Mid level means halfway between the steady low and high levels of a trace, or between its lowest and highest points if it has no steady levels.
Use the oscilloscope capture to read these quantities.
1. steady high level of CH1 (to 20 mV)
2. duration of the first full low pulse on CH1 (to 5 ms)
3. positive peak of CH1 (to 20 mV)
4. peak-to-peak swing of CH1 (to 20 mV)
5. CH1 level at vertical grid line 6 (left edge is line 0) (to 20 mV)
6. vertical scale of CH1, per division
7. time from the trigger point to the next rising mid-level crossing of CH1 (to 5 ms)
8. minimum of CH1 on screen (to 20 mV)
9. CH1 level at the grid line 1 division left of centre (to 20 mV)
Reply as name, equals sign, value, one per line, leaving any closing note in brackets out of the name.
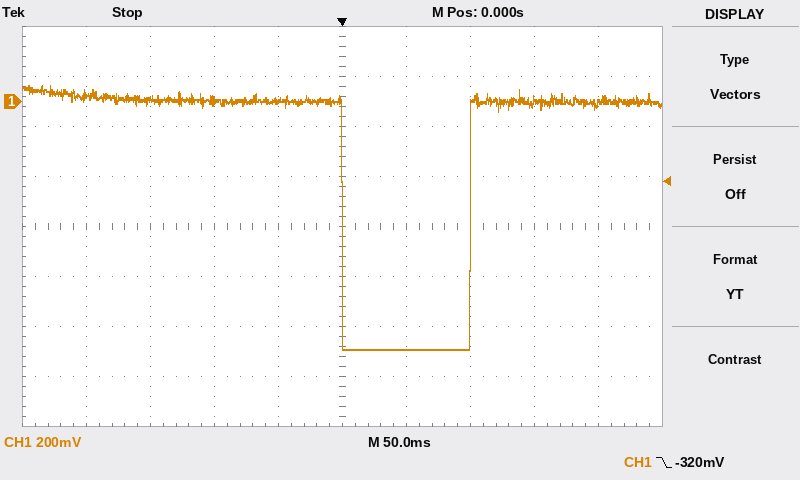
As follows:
steady high level of CH1 = 0 mV
duration of the first full low pulse on CH1 = 100 ms
positive peak of CH1 = 60 mV
peak-to-peak swing of CH1 = 1.06 V
CH1 level at vertical grid line 6 (left edge is line 0) = -1.00 V
vertical scale of CH1, per division = 200 mV
time from the trigger point to the next rising mid-level crossing of CH1 = 100 ms
minimum of CH1 on screen = -1.00 V
CH1 level at the grid line 1 division left of centre = 0 mV
